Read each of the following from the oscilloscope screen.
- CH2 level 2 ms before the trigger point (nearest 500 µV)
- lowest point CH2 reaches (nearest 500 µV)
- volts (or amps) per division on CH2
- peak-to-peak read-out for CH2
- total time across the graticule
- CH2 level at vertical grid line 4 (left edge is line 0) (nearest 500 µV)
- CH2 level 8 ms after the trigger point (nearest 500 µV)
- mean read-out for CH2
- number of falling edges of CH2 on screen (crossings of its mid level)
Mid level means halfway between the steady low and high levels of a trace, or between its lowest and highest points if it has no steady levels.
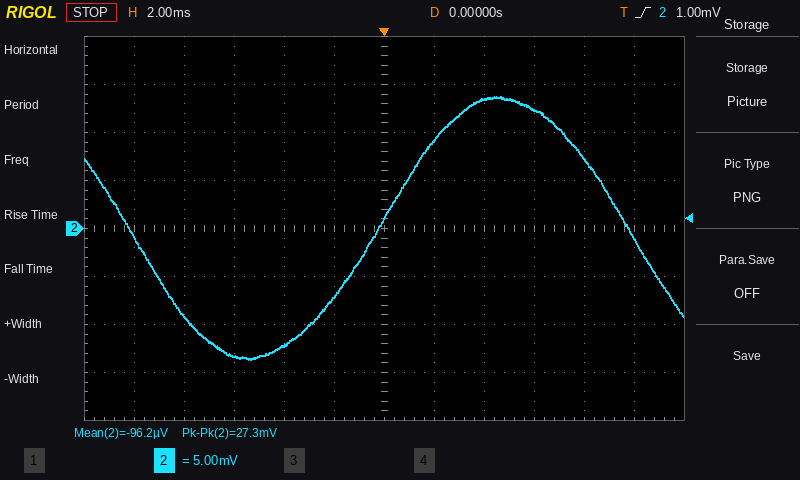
-7.0 mV
-13.5 mV
5 mV
27.3 mV
24 ms
-12.0 mV
7.5 mV
-96.2 µV
2
